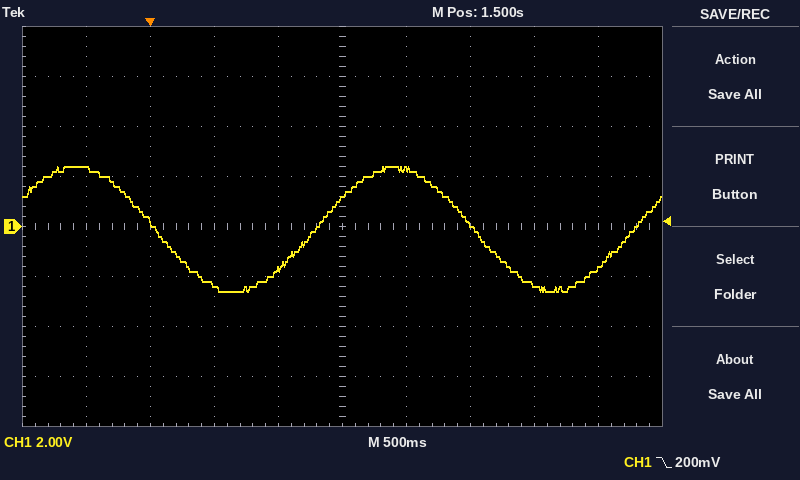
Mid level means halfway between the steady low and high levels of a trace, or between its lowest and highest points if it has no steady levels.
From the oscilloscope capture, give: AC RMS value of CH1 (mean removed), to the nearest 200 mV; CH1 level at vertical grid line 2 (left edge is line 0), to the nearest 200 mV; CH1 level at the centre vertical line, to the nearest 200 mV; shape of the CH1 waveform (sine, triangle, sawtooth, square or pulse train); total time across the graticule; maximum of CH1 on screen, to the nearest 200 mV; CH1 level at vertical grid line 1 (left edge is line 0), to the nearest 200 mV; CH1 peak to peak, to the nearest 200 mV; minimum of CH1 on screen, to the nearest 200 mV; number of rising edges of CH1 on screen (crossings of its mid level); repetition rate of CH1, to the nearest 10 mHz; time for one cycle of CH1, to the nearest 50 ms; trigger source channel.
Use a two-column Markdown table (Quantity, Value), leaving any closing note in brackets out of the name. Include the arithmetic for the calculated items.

| Quantity | Value |
|---|---|
| AC RMS value of CH1 (mean removed), to the nearest 200 mV | 5.0 V / (2√2) ≈ 1.8 V |
| CH1 level at vertical grid line 2 (left edge is line 0), to the nearest 200 mV | 200 mV |
| CH1 level at the centre vertical line, to the nearest 200 mV | 1.2 V |
| shape of the CH1 waveform | sine |
| total time across the graticule | 5 s |
| maximum of CH1 on screen, to the nearest 200 mV | 2.4 V |
| CH1 level at vertical grid line 1 (left edge is line 0), to the nearest 200 mV | 2.4 V |
| CH1 peak to peak, to the nearest 200 mV | 2.4 V − (-2.6 V) = 5.0 V |
| minimum of CH1 on screen, to the nearest 200 mV | -2.6 V |
| number of rising edges of CH1 on screen | 2 |
| repetition rate of CH1, to the nearest 10 mHz | 1 / 2.50 s ≈ 400 mHz |
| time for one cycle of CH1, to the nearest 50 ms | 2.50 s |
| trigger source channel | CH1 |
